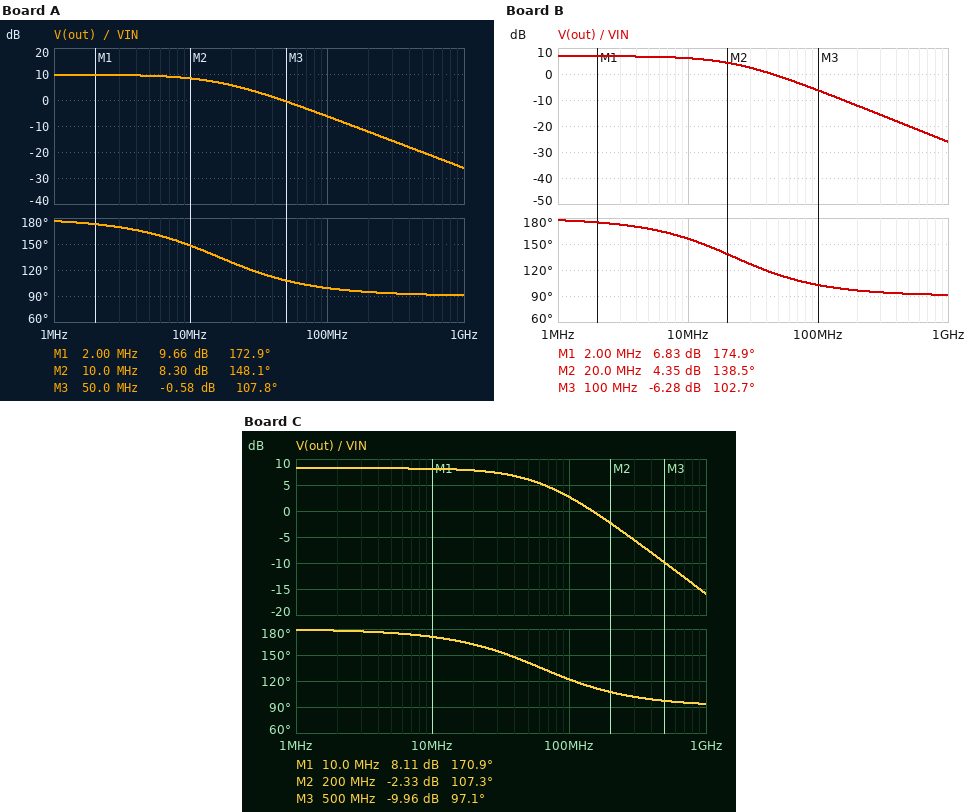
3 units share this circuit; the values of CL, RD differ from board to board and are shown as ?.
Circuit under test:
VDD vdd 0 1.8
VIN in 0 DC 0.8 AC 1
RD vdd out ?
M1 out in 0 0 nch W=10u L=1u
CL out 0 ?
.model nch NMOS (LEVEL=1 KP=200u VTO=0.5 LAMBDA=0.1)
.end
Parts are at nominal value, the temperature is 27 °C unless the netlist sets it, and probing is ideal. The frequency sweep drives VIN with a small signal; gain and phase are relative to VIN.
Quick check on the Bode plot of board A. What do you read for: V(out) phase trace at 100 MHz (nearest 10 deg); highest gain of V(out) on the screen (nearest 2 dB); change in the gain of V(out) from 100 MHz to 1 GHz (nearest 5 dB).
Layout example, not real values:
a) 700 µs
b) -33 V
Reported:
a) 100 deg
b) 10 dB
c) -20 dB
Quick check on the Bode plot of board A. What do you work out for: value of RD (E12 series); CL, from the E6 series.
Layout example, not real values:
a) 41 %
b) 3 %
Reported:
a) 4.7 kΩ
b) 2.2 pF
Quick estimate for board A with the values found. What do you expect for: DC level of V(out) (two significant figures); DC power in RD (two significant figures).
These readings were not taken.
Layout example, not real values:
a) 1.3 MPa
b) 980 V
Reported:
a) 1.3 V
b) 49 µW
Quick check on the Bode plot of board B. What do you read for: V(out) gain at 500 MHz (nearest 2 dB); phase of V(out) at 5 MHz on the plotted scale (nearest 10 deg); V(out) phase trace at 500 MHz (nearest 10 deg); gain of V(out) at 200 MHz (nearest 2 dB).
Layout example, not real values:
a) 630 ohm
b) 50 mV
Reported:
a) -20 dB
b) 170 deg
c) 90 deg
d) -12 dB
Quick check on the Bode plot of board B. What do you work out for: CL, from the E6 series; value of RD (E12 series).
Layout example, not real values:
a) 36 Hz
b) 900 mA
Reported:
a) 2.2 pF
b) 3.3 kΩ
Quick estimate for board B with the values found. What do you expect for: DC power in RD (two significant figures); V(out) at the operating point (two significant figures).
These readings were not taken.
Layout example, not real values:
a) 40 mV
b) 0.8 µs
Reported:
a) 35 µW
b) 1.5 V
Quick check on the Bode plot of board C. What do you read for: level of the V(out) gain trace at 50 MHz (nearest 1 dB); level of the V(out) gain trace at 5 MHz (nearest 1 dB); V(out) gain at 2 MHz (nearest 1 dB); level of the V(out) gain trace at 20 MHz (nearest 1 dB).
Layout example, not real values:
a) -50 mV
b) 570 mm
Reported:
a) 6 dB
b) 8 dB
c) 8 dB
d) 8 dB
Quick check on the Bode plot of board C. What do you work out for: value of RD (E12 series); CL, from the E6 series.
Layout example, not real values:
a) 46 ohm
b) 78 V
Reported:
a) 3.9 kΩ
b) 680 fF
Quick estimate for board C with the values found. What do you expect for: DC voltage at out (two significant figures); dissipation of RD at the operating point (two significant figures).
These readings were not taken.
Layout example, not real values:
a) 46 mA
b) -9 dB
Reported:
a) 1.4 V
b) 41 µW
